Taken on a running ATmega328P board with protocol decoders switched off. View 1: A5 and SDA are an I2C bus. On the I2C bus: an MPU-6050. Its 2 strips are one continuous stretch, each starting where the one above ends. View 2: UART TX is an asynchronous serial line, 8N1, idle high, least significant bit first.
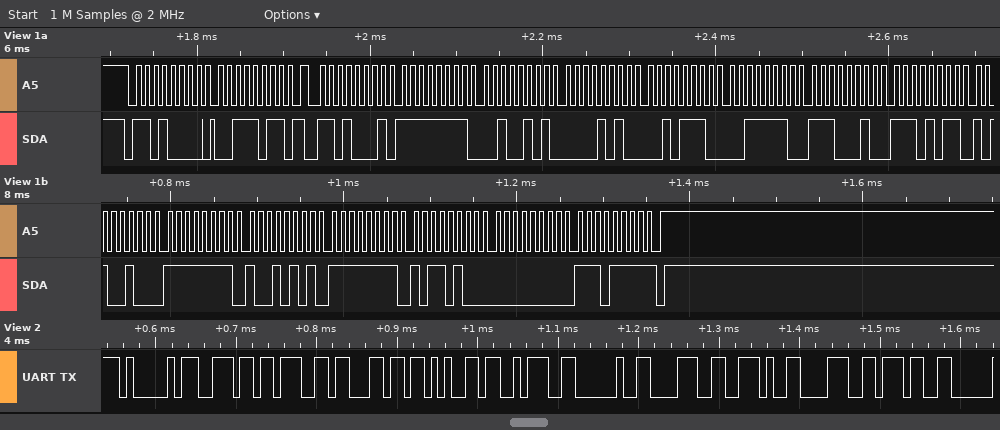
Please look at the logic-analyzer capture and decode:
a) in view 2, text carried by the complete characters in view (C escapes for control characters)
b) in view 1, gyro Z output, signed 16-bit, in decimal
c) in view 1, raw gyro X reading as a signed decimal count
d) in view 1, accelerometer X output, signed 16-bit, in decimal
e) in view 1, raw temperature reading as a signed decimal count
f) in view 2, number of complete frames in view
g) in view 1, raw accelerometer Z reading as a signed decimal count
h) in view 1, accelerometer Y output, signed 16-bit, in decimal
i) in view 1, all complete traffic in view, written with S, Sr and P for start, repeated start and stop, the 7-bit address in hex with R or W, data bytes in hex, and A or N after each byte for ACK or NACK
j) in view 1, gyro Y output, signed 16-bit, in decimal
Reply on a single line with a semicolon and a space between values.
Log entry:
"Angle: 8.87"; 239; -107; -219; -5212; 11; 16098; 2606; S 68W A 3B A Sr 68R A FF A 25 A 0A A 2E A 3E A E2 A EB A A4 A FF A 95 A FF A B4 A 00 A EF N P; -76
